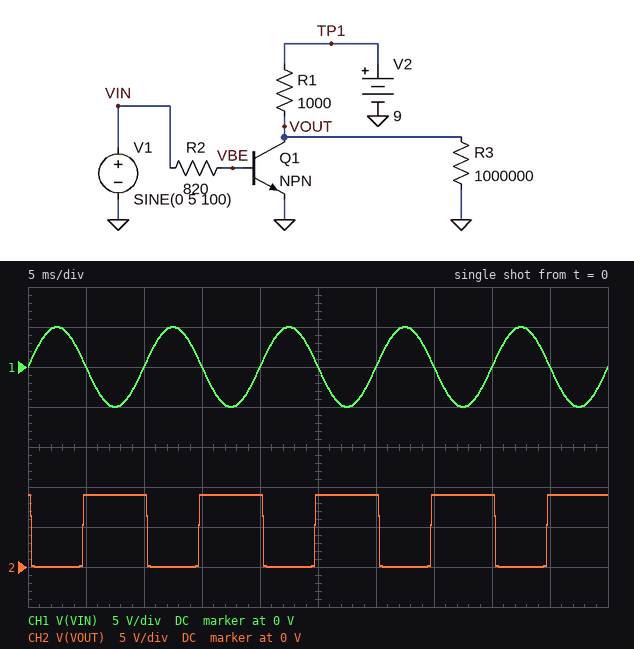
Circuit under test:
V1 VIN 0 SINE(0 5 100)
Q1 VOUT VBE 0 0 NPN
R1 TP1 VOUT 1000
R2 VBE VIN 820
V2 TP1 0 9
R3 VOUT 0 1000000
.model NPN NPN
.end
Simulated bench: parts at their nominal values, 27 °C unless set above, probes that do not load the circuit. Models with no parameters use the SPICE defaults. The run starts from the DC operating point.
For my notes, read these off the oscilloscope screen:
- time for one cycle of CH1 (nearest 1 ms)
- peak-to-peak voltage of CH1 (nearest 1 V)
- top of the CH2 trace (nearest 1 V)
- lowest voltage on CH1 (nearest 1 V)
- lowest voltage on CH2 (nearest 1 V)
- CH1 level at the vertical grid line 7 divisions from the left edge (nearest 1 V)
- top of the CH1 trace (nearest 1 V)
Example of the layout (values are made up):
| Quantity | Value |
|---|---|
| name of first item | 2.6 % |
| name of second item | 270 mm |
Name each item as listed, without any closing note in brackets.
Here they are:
| Quantity | Value |
|---|---|
| time for one cycle of CH1 | 10 ms |
| peak-to-peak voltage of CH1 | 10 V |
| top of the CH2 trace | 9 V |
| lowest voltage on CH1 | -5 V |
| lowest voltage on CH2 | 0 V |
| CH1 level at the vertical grid line 7 divisions from the left edge | 0 V |
| top of the CH1 trace | 5 V |
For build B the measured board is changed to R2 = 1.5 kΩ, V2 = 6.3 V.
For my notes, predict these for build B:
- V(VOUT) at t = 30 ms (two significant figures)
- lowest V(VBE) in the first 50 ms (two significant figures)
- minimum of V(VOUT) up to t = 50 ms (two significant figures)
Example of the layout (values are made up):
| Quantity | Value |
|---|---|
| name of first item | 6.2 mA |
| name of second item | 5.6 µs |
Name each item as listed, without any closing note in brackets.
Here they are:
| Quantity | Value |
|---|---|
| V(VOUT) at t = 30 ms | 6.3 V |
| lowest V(VBE) in the first 50 ms | -5.0 V |
| minimum of V(VOUT) up to t = 50 ms | 38 mV |
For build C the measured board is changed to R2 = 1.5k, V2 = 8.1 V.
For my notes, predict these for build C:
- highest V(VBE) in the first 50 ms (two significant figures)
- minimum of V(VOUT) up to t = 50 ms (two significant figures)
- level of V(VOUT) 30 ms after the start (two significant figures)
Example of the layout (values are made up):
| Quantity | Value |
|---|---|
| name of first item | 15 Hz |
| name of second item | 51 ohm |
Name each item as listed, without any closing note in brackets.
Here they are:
| Quantity | Value |
|---|---|
| highest V(VBE) in the first 50 ms | 840 mV |
| minimum of V(VOUT) up to t = 50 ms | 42 mV |
| level of V(VOUT) 30 ms after the start | 8.1 V |
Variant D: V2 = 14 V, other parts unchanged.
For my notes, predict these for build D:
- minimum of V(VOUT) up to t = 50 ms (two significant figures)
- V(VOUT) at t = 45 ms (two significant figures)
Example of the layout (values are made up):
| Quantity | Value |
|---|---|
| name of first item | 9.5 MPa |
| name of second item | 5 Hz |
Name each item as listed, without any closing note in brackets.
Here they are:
| Quantity | Value |
|---|---|
| minimum of V(VOUT) up to t = 50 ms | 41 mV |
| V(VOUT) at t = 45 ms | 14 V |
